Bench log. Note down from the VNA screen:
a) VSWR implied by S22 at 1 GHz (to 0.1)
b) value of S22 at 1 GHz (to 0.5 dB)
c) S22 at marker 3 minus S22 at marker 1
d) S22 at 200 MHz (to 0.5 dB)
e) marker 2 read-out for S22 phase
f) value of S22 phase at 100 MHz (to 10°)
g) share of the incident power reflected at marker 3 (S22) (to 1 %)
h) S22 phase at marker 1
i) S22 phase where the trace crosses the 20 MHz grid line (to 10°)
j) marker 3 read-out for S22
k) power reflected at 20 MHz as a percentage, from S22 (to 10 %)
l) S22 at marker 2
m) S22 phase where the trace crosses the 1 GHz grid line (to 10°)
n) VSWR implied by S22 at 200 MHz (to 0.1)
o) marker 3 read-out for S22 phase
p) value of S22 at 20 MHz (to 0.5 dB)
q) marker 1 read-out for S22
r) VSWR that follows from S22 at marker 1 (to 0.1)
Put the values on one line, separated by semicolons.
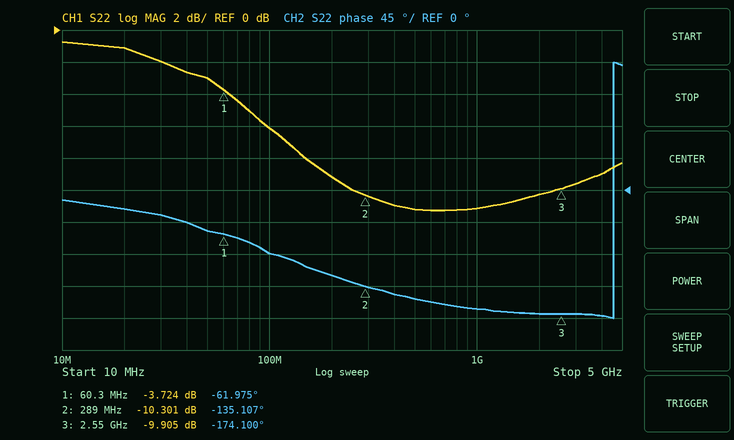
1.8; -11.0 dB; -6.181 dB; -9.0 dB; -135.107°; -90°; 10 %; -61.975°; -30°; -9.905 dB; 80 %; -10.301 dB; -170°; 2.1; -174.100°; -1.0 dB; -3.724 dB; 4.7
